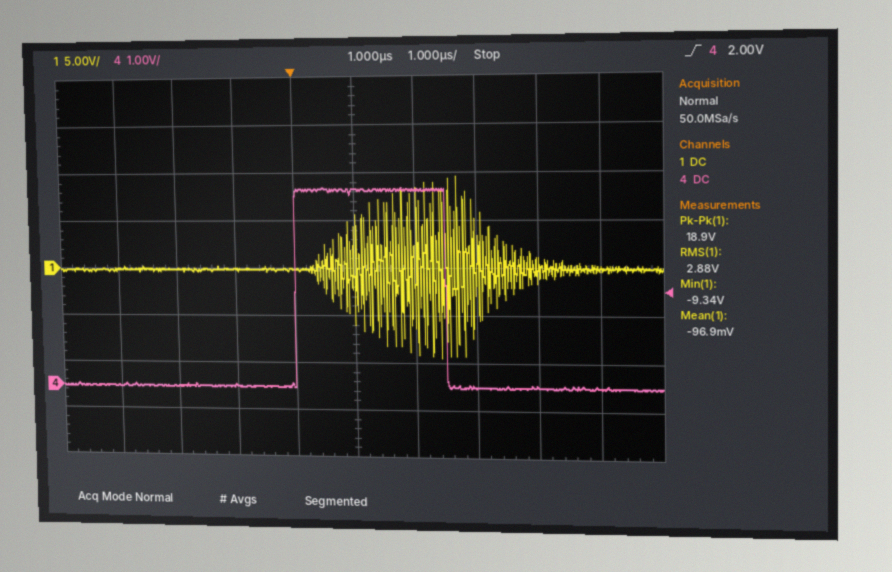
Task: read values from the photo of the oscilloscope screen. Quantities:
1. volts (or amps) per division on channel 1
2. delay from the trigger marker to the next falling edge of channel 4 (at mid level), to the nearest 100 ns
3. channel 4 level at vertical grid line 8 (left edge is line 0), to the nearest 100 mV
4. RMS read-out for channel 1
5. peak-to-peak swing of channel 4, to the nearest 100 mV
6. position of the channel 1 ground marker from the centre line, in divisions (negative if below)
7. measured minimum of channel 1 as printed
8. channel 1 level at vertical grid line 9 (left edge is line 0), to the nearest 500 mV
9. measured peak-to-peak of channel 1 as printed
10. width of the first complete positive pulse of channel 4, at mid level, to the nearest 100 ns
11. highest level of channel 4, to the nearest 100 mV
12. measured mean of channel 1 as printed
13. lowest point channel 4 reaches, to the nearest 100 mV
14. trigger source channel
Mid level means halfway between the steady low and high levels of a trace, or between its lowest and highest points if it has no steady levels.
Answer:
5 V
2.5 µs
0.0 V
2.88 V
4.2 V
0.0 div
-9.34 V
0.0 V
18.9 V
2.5 µs
4.2 V
-96.9 mV
0.0 V
channel 4
